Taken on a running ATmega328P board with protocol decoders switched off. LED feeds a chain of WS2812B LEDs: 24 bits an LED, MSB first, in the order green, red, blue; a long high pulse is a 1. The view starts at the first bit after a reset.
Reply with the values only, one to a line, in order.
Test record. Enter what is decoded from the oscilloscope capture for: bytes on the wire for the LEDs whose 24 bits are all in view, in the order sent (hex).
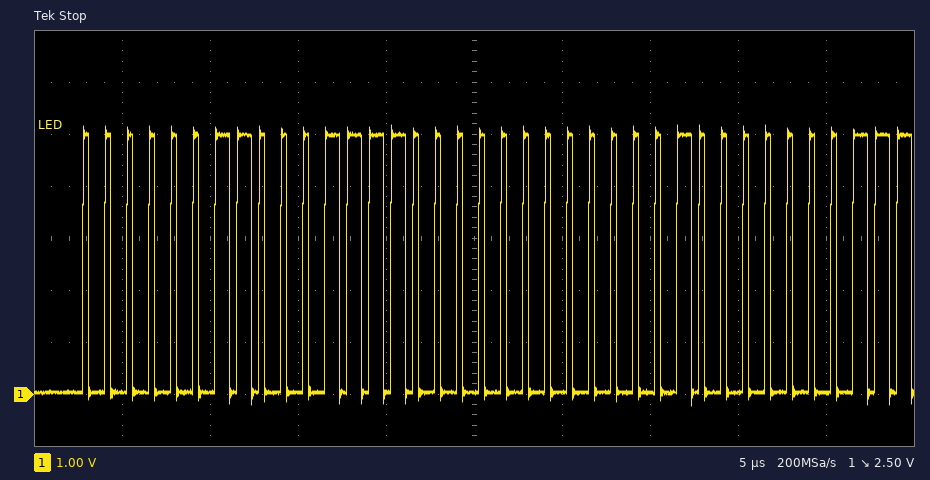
03 1E 00
